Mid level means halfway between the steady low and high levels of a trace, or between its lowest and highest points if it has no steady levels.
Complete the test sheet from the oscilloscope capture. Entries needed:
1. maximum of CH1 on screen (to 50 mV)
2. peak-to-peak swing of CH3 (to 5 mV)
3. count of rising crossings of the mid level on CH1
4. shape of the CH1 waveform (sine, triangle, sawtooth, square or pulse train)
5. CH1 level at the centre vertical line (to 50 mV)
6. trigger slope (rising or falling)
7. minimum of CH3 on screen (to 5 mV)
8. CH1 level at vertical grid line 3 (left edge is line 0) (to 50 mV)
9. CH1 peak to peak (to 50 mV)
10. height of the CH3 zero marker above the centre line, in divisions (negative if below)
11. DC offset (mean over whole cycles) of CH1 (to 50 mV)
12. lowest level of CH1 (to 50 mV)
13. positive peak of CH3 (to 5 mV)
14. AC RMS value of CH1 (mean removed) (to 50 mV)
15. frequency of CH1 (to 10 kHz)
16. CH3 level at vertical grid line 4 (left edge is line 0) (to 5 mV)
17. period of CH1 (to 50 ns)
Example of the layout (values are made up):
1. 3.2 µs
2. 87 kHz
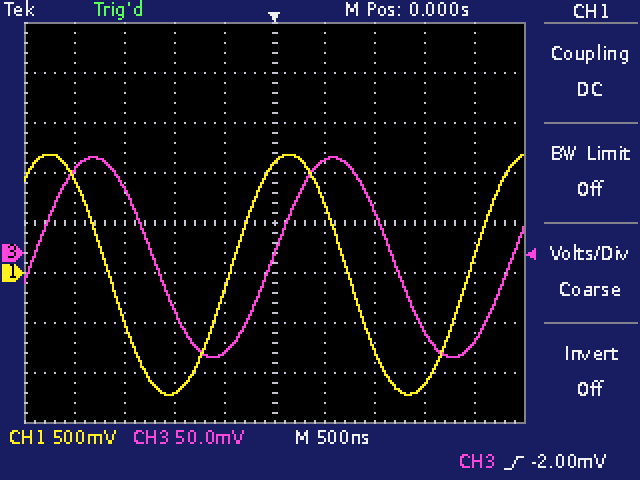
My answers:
1. 1.20 V
2. 200 mV
3. 2
4. sine
5. 1.10 V
6. rising
7. -105 mV
8. -1.20 V
9. 2.40 V
10. -0.6 div
11. 0 mV
12. -1.20 V
13. 95 mV
14. 850 mV
15. 420 kHz
16. -100 mV
17. 2.40 µs
